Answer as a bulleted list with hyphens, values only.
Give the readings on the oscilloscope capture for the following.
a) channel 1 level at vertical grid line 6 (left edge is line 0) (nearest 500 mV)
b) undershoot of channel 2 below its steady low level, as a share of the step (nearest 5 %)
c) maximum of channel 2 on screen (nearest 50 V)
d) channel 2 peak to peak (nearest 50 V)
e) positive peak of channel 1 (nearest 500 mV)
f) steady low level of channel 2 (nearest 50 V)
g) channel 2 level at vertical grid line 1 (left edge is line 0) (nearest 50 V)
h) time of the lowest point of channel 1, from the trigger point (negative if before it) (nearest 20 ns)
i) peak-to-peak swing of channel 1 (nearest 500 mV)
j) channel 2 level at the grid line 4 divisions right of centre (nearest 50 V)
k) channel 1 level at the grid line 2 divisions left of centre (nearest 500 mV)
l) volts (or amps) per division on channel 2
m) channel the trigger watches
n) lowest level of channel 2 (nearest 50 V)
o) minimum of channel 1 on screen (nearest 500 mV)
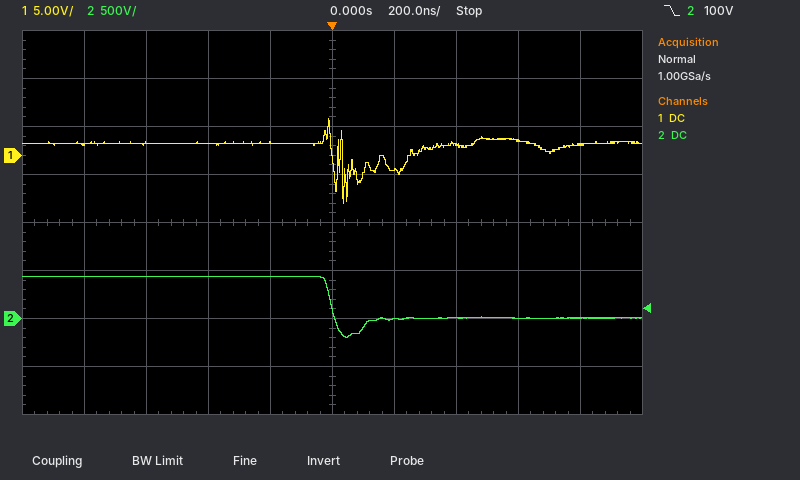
- -1.5 V
- 45 %
- 450 V
- 650 V
- 4.0 V
- 0 V
- 450 V
- +40 ns
- 9.0 V
- 0 V
- 1.0 V
- 500 V
- channel 2
- -200 V
- -5.0 V
